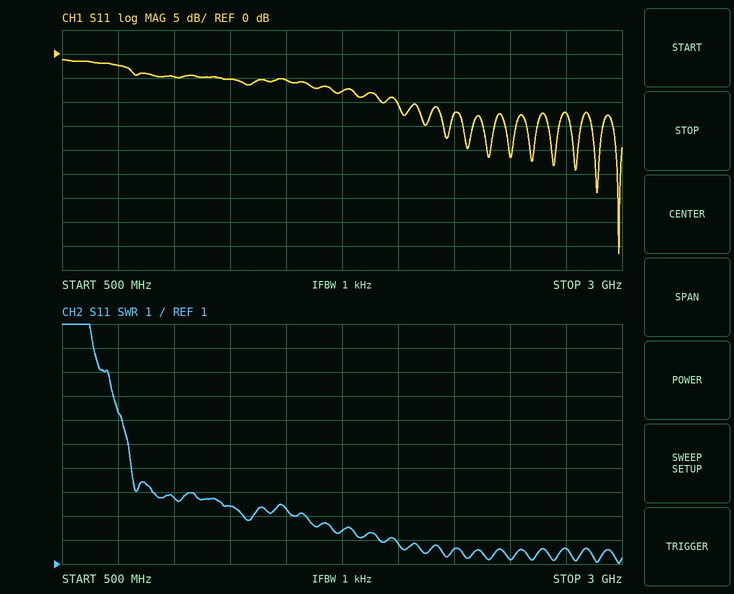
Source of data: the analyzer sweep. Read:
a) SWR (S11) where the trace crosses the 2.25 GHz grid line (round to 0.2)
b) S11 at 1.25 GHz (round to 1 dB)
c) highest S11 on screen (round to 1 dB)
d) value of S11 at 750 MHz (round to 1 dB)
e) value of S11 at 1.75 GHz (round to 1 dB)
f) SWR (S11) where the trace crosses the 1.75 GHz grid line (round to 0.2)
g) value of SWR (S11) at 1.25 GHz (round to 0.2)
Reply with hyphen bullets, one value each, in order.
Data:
- 1.6
- -5 dB
- -1 dB
- -2 dB
- -8 dB
- 2.4
- 3.4
